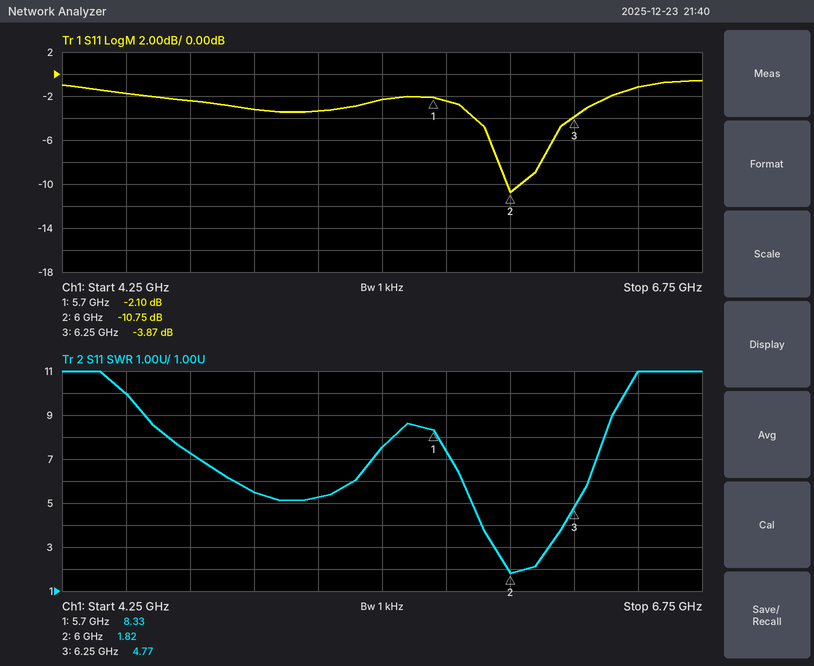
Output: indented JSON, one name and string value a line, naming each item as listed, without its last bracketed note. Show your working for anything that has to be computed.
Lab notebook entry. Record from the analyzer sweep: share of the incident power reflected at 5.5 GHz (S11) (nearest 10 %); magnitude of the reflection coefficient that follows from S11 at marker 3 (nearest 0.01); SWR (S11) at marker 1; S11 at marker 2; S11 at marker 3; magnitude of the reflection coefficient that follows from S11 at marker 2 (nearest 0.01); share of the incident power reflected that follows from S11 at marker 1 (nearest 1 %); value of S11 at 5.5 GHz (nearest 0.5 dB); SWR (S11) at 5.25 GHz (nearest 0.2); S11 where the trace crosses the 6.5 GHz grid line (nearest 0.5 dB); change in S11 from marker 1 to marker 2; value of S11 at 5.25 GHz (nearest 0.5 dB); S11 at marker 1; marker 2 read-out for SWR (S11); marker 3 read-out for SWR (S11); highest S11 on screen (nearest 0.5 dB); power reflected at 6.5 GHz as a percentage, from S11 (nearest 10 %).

{
  "share of the incident power reflected at 5.5 GHz (S11)": "10^(-2.5/10) ≈ 56.2 %, so 60 % to the nearest 10 %",
  "magnitude of the reflection coefficient that follows from S11 at marker 3": "10^(-3.87/20) ≈ 0.64",
  "SWR (S11) at marker 1": "8.33",
  "S11 at marker 2": "-10.75 dB",
  "S11 at marker 3": "-3.87 dB",
  "magnitude of the reflection coefficient that follows from S11 at marker 2": "10^(-10.75/20) ≈ 0.29",
  "share of the incident power reflected that follows from S11 at marker 1": "10^(-2.1/10) ≈ 62 %",
  "value of S11 at 5.5 GHz": "-2.5 dB",
  "SWR (S11) at 5.25 GHz": "5.2",
  "S11 where the trace crosses the 6.5 GHz grid line": "-1.0 dB",
  "change in S11 from marker 1 to marker 2": "-10.75 − (-2.1) = -8.65 dB",
  "value of S11 at 5.25 GHz": "-3.5 dB",
  "S11 at marker 1": "-2.10 dB",
  "marker 2 read-out for SWR": "1.82",
  "marker 3 read-out for SWR": "4.77",
  "highest S11 on screen": "-0.5 dB",
  "power reflected at 6.5 GHz as a percentage, from S11": "10^(-1/10) ≈ 79.4 %, so 80 % to the nearest 10 %"
}
